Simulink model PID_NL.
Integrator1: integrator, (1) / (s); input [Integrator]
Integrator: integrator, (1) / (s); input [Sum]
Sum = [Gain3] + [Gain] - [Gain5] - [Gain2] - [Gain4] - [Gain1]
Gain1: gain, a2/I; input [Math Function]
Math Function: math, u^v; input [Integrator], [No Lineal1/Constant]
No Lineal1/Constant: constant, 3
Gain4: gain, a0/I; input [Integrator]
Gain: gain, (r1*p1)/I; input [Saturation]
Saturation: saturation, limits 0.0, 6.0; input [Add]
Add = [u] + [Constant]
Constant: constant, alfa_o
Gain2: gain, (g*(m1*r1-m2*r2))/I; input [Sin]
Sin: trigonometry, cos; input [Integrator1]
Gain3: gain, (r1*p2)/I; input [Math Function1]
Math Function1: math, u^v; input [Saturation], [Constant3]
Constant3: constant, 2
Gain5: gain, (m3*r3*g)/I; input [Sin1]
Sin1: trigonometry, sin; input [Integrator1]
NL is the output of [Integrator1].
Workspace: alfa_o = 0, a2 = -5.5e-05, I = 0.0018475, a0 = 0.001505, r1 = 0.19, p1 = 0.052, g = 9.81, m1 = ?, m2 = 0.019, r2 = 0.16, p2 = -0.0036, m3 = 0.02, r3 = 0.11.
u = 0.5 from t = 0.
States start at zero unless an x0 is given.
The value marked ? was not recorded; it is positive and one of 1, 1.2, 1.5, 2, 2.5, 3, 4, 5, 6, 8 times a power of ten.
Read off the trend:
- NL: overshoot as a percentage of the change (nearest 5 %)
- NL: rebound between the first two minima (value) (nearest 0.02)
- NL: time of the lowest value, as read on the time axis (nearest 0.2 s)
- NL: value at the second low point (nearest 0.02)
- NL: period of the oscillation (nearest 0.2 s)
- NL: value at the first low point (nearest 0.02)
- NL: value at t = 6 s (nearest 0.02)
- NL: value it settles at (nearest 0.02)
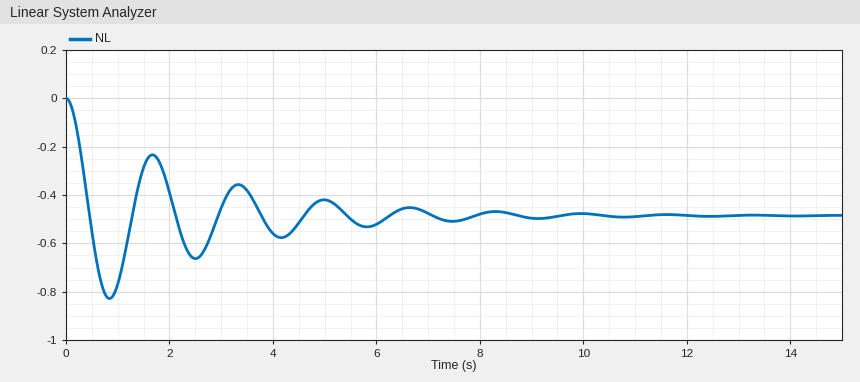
70 %
-0.24
0.8 s
-0.66
1.6 s
-0.82
-0.52
-0.48
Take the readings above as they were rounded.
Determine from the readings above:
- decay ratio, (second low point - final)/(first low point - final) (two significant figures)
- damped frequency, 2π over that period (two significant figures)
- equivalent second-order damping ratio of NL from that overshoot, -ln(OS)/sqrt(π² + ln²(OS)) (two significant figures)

0.53
3.9 rad/s
0.11
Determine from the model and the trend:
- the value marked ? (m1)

0.025
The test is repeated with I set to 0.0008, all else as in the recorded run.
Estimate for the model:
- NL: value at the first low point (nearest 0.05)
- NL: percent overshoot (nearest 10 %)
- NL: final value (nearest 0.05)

-0.80
60 %
-0.50
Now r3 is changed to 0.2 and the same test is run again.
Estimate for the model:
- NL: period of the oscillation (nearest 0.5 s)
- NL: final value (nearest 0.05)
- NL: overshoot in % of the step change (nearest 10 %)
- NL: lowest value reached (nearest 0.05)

1.5 s
-0.30
80 %
-0.50
